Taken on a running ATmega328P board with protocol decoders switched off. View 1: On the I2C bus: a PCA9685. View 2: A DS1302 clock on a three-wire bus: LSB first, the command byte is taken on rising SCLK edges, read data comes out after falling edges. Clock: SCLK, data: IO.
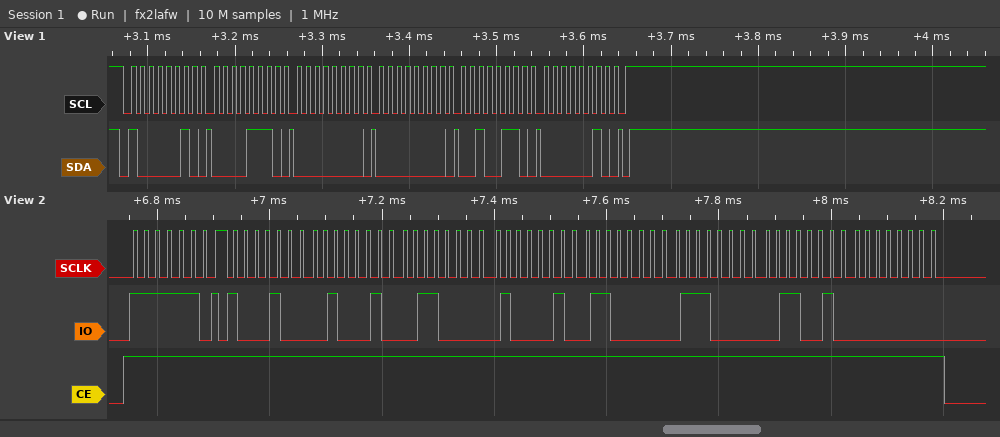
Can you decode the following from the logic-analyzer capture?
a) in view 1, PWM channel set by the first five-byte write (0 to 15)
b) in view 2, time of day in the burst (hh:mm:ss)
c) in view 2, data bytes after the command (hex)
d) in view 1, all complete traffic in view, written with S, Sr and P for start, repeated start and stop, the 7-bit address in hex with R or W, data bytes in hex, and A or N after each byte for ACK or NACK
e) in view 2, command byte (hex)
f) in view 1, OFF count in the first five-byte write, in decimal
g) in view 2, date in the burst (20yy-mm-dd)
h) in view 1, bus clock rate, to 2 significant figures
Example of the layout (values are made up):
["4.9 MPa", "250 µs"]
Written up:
["2", "06:22:11", "11 22 06 21 03 07 26 00", "S 41W A 0E A 00 A 00 A 26 A 02 A P", "0xBF", "550", "2026-03-21", "100 kHz"]
